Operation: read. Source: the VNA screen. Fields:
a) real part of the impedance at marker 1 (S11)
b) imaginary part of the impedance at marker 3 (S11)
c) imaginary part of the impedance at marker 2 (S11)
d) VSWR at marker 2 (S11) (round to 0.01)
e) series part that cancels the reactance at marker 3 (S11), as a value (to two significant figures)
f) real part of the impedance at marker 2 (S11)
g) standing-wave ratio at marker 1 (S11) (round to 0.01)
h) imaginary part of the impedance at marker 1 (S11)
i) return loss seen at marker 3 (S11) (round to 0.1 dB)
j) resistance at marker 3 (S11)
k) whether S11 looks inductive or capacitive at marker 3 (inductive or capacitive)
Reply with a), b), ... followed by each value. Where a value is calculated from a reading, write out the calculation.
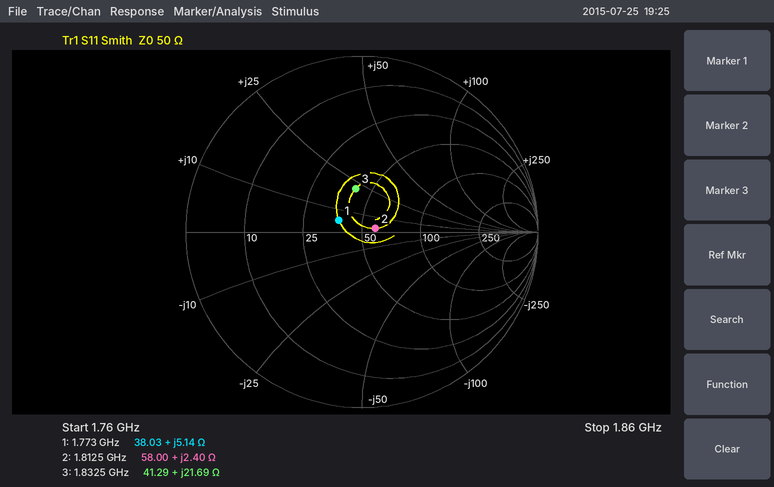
a) 38.03 Ω
b) +21.69 Ω
c) +2.40 Ω
d) 1.17
e) C = 1/(2π × 1.8325 GHz × 21.69 Ω) ≈ 4.0 pF
f) 58.00 Ω
g) 1.35
h) +5.14 Ω
i) 12.1 dB
j) 41.29 Ω
k) inductive
